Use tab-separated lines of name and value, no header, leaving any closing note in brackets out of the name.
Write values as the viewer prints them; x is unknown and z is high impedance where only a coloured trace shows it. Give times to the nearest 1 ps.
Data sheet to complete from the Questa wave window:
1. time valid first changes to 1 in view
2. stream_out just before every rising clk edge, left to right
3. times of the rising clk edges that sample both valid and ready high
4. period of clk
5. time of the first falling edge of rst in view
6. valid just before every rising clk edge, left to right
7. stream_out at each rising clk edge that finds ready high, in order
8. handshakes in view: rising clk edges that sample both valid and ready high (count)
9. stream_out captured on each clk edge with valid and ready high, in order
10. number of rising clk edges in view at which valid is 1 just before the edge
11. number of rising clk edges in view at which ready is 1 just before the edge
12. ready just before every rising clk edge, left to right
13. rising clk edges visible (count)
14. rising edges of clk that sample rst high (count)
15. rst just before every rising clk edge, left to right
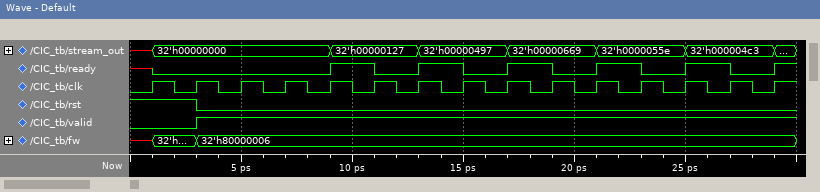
time valid first changes to 1 in view	3 ps
stream_out just before every rising clk edge, left to right	x, 32'h00000000, 32'h00000000, 32'h00000000, 32'h00000000, 32'h00000127, 32'h00000127, 32'h00000497, 32'h00000497, 32'h00000669, 32'h00000669, 32'h0000055e, 32'h0000055e, 32'h000004c3, 32'h000004c3
times of the rising clk edges that sample both valid and ready high	11 ps, 15 ps, 19 ps, 23 ps, 27 ps
period of clk	2 ps
time of the first falling edge of rst in view	3 ps
valid just before every rising clk edge, left to right	0 0 1 1 1 1 1 1 1 1 1 1 1 1 1
stream_out at each rising clk edge that finds ready high, in order	32'h00000127, 32'h00000497, 32'h00000669, 32'h0000055e, 32'h000004c3
handshakes in view: rising clk edges that sample both valid and ready high	5
stream_out captured on each clk edge with valid and ready high, in order	32'h00000127, 32'h00000497, 32'h00000669, 32'h0000055e, 32'h000004c3
number of rising clk edges in view at which valid is 1 just before the edge	13
number of rising clk edges in view at which ready is 1 just before the edge	5
ready just before every rising clk edge, left to right	x 0 0 0 0 1 0 1 0 1 0 1 0 1 0
rising clk edges visible	15
rising edges of clk that sample rst high	2
rst just before every rising clk edge, left to right	1 1 0 0 0 0 0 0 0 0 0 0 0 0 0
